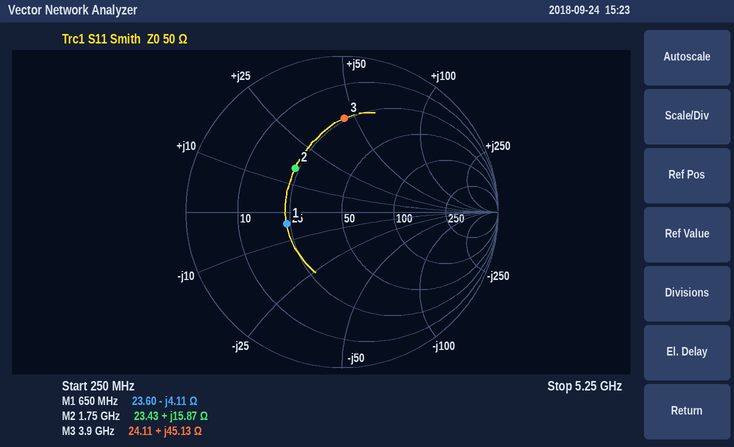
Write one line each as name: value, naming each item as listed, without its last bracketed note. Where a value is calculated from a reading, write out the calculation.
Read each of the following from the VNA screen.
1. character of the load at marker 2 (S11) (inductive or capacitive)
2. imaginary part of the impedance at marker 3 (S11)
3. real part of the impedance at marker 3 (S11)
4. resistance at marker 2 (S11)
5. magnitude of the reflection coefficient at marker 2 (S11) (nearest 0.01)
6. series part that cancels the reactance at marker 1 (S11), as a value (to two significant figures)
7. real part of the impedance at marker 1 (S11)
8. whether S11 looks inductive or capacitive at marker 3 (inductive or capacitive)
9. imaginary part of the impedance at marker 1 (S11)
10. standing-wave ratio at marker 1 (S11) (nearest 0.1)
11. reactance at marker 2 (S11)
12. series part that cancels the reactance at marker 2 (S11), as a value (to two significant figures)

character of the load at marker 2 (S11): inductive
imaginary part of the impedance at marker 3: +45.13 Ω
real part of the impedance at marker 3: 24.11 Ω
resistance at marker 2: 23.43 Ω
magnitude of the reflection coefficient at marker 2 (S11): 0.41
series part that cancels the reactance at marker 1 (S11), as a value: L = 4.11 Ω/(2π × 650 MHz) ≈ 1.0 nH
real part of the impedance at marker 1: 23.60 Ω
whether S11 looks inductive or capacitive at marker 3: inductive
imaginary part of the impedance at marker 1: -4.11 Ω
standing-wave ratio at marker 1 (S11): 2.1
reactance at marker 2: +15.87 Ω
series part that cancels the reactance at marker 2 (S11), as a value: C = 1/(2π × 1.75 GHz × 15.87 Ω) ≈ 5.7 pF
